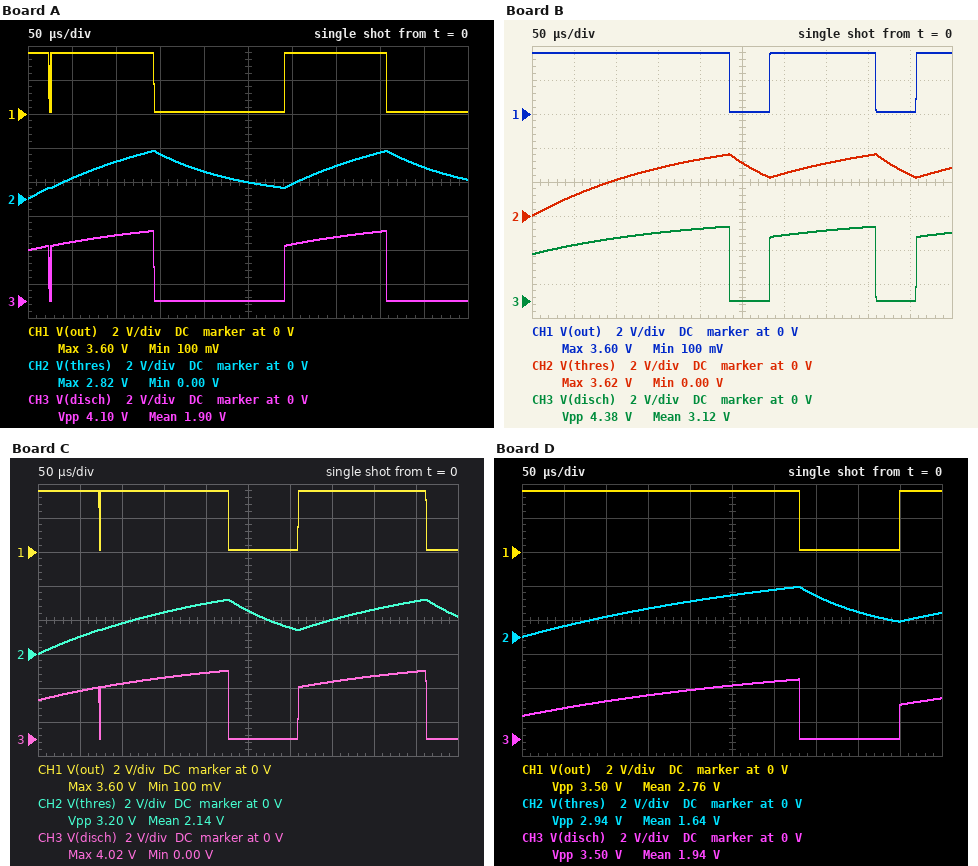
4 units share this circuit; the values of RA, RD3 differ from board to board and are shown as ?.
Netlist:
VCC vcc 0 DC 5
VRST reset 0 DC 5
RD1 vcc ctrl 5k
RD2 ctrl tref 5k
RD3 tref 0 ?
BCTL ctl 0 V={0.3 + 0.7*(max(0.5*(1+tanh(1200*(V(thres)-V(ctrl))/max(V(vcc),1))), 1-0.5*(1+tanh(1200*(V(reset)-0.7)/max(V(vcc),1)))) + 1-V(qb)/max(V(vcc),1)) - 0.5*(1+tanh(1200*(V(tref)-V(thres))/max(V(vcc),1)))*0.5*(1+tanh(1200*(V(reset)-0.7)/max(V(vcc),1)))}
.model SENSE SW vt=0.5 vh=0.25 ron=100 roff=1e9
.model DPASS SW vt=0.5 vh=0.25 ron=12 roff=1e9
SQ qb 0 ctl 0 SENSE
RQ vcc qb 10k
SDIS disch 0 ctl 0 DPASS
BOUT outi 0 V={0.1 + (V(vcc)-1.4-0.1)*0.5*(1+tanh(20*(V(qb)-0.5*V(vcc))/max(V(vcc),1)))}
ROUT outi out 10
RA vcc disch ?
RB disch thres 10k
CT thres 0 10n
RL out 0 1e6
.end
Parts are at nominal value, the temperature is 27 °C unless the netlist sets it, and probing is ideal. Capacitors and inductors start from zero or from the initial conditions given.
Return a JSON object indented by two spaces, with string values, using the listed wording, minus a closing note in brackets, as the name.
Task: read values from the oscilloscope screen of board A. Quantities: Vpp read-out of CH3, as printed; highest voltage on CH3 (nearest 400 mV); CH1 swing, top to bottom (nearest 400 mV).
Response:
{
  "Vpp read-out of CH3, as printed": "4.10 V",
  "highest voltage on CH3": "4.0 V",
  "CH1 swing, top to bottom": "3.6 V"
}
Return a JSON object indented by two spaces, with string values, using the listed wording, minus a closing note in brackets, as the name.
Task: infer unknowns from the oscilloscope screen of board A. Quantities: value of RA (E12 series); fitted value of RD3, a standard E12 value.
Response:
{
  "value of RA": "6.8 kΩ",
  "fitted value of RD3, a standard E12 value": "1.5 kΩ"
}
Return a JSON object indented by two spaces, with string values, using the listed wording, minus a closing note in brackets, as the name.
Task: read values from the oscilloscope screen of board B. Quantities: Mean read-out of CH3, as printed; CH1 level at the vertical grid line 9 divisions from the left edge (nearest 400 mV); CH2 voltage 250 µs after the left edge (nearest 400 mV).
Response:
{
  "Mean read-out of CH3, as printed": "3.12 V",
  "CH1 level at the vertical grid line 9 divisions from the left edge": "0 V",
  "CH2 voltage 250 µs after the left edge": "3.2 V"
}
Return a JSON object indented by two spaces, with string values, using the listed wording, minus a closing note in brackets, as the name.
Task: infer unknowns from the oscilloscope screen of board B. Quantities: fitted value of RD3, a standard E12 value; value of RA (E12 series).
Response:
{
  "fitted value of RD3, a standard E12 value": "8.2 kΩ",
  "value of RA": "8.2 kΩ"
}
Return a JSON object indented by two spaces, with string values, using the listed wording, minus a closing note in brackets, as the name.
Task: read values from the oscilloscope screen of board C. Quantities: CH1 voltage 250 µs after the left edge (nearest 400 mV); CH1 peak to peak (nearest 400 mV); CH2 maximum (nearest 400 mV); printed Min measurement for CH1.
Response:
{
  "CH1 voltage 250 µs after the left edge": "0 V",
  "CH1 peak to peak": "3.6 V",
  "CH2 maximum": "3.2 V",
  "printed Min measurement for CH1": "100 mV"
}
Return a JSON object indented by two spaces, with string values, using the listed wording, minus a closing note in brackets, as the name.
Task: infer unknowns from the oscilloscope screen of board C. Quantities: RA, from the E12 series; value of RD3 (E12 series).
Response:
{
  "RA, from the E12 series": "12 kΩ",
  "value of RD3": "3.9 kΩ"
}
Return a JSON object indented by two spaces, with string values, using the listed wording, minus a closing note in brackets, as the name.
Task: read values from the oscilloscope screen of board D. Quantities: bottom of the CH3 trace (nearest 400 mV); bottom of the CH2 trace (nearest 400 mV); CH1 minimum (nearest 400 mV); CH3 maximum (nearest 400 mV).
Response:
{
  "bottom of the CH3 trace": "0 V",
  "bottom of the CH2 trace": "0 V",
  "CH1 minimum": "0 V",
  "CH3 maximum": "3.6 V"
}
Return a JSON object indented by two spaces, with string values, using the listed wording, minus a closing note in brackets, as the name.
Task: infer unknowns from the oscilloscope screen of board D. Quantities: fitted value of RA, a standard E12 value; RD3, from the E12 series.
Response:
{
  "fitted value of RA, a standard E12 value": "27 kΩ",
  "RD3, from the E12 series": "2.2 kΩ"
}
